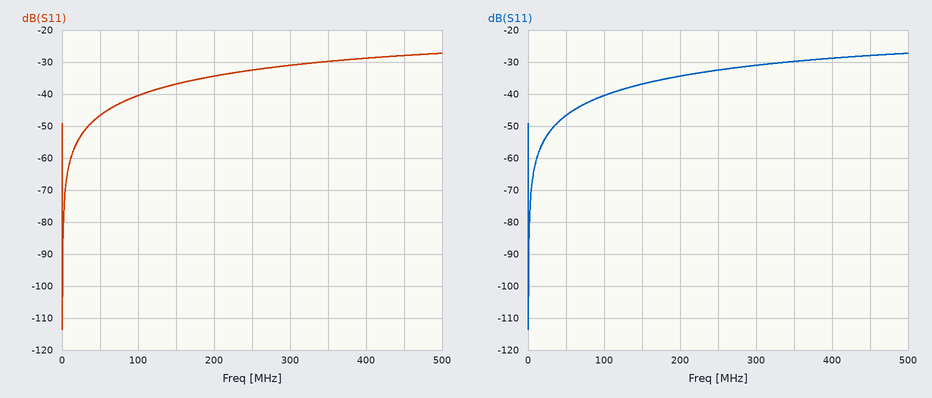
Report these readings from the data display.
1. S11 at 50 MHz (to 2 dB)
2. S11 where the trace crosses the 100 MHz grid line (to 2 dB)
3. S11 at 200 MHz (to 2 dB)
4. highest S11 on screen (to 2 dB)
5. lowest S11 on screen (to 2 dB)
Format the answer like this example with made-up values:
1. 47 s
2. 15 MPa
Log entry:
1. -46 dB
2. -40 dB
3. -34 dB
4. -28 dB
5. -114 dB
